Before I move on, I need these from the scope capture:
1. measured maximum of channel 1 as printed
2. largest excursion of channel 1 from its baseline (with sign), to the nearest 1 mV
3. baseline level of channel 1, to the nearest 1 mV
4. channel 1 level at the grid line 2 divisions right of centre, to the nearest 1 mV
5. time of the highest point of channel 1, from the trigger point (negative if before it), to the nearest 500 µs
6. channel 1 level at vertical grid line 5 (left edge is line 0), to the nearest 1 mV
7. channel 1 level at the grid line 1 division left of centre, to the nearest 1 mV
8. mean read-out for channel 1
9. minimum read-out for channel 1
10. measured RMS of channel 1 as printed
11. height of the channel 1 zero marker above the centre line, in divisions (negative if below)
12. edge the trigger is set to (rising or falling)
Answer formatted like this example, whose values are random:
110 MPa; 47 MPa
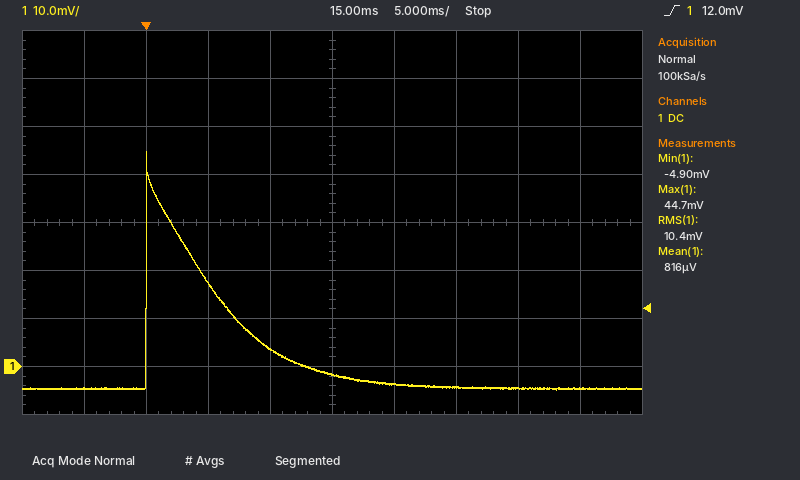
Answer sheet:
44.7 mV; +49 mV; -5 mV; -4 mV; 0.0 ms; -2 mV; 4 mV; 816 µV; -4.90 mV; 10.4 mV; -3.0 div; rising
